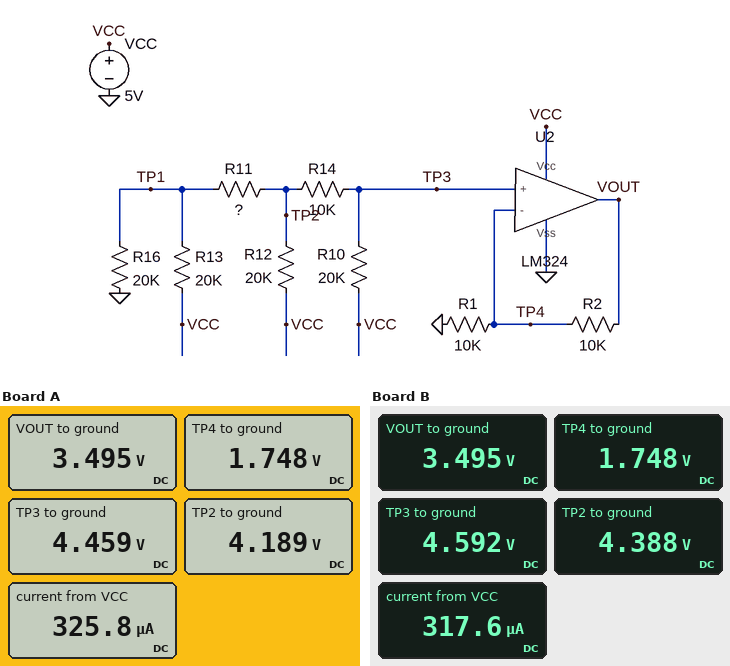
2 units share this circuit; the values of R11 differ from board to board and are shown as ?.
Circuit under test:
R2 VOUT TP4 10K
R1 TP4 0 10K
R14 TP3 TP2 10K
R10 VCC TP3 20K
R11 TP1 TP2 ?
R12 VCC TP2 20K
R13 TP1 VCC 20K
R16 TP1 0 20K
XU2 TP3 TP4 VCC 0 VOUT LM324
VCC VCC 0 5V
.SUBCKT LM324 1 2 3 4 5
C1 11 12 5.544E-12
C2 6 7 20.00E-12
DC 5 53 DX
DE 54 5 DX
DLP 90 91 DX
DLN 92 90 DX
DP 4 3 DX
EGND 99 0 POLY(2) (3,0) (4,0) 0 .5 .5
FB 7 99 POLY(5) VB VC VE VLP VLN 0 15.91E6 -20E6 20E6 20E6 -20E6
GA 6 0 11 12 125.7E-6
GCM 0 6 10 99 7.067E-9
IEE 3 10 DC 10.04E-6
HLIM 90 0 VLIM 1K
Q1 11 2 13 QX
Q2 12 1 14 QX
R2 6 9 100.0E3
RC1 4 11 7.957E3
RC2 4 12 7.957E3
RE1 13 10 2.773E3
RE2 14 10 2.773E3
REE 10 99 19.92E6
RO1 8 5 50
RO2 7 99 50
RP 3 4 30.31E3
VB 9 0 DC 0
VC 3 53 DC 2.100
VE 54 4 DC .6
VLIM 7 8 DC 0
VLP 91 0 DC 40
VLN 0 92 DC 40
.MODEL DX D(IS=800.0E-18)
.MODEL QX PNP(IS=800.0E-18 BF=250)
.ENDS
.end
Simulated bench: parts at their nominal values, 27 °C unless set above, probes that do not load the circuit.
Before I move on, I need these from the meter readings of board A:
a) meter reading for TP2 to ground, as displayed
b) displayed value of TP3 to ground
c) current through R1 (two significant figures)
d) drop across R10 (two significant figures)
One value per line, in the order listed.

4.189 V
4.459 V
170 µA
540 mV
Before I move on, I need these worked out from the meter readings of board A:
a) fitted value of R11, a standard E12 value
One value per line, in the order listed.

15 kΩ
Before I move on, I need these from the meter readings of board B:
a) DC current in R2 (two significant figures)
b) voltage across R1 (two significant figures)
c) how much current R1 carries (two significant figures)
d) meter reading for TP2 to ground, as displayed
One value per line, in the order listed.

170 µA
1.7 V
170 µA
4.388 V
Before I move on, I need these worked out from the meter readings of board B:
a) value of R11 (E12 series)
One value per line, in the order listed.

27 kΩ
